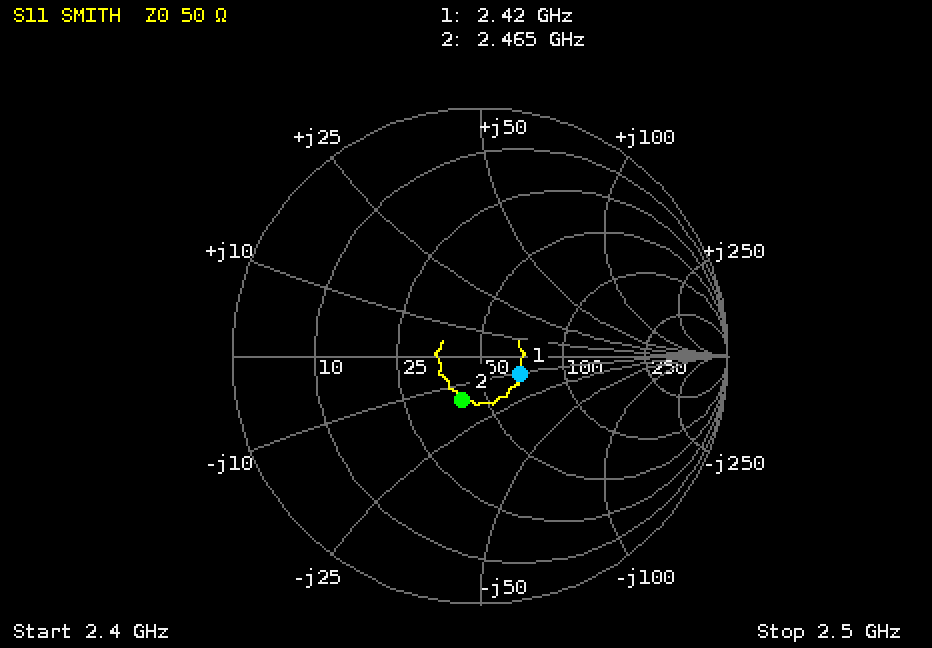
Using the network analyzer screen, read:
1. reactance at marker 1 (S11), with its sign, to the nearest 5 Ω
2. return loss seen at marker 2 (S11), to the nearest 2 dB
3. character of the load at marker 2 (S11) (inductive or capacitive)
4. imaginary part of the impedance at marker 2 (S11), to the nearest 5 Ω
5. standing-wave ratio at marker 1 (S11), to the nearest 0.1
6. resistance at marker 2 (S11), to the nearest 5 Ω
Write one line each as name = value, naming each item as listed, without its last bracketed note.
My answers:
reactance at marker 1 (S11), with its sign, to the nearest 5 Ω = -10 Ω
return loss seen at marker 2 (S11), to the nearest 2 dB = 14 dB
character of the load at marker 2 (S11) = capacitive
imaginary part of the impedance at marker 2 (S11), to the nearest 5 Ω = -15 Ω
standing-wave ratio at marker 1 (S11), to the nearest 0.1 = 1.4
resistance at marker 2 (S11), to the nearest 5 Ω = 40 Ω
